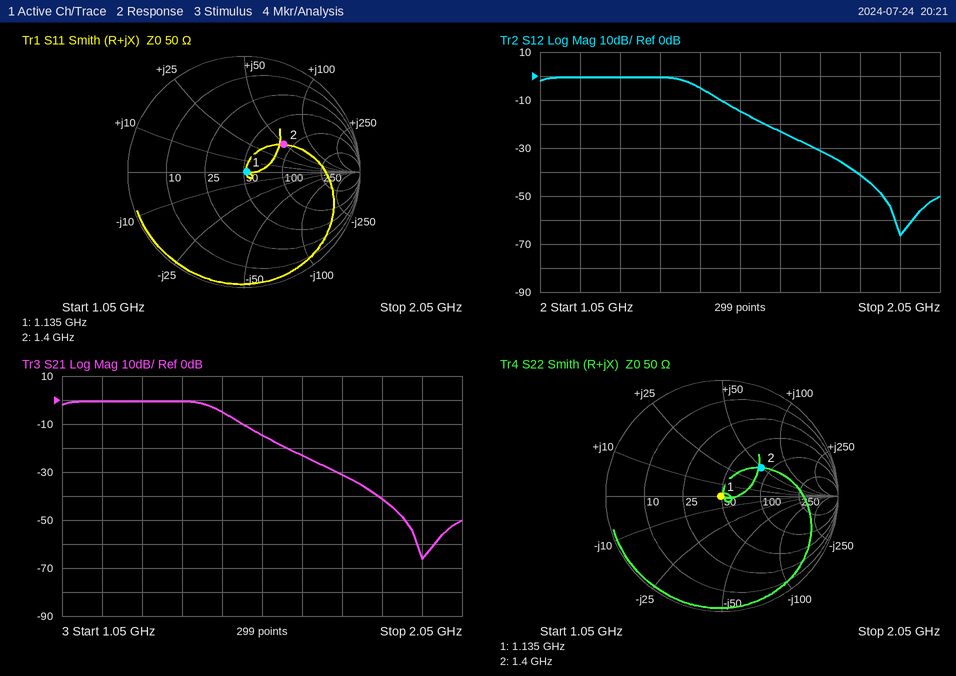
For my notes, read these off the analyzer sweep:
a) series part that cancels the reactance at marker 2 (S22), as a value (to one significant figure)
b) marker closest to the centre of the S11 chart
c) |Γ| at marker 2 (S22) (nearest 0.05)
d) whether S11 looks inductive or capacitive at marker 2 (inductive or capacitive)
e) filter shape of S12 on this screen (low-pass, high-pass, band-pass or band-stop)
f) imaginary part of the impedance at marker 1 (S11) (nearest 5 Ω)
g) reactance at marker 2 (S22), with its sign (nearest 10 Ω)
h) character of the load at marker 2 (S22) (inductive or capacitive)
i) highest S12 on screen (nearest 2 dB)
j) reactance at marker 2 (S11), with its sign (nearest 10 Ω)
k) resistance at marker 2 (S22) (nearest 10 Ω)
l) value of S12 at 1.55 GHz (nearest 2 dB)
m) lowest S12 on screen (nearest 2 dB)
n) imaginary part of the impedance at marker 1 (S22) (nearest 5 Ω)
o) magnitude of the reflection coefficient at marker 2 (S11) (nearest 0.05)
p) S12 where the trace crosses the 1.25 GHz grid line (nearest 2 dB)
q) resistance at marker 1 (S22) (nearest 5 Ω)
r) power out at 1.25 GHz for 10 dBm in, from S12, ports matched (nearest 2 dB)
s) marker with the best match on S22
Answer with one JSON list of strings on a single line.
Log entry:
["2 pF", "marker 1", "0.40", "inductive", "low-pass", "0 Ω", "+50 Ω", "inductive", "0 dB", "+50 Ω", "80 Ω", "-14 dB", "-66 dB", "0 Ω", "0.40", "0 dB", "50 Ω", "10 dBm", "marker 1"]
